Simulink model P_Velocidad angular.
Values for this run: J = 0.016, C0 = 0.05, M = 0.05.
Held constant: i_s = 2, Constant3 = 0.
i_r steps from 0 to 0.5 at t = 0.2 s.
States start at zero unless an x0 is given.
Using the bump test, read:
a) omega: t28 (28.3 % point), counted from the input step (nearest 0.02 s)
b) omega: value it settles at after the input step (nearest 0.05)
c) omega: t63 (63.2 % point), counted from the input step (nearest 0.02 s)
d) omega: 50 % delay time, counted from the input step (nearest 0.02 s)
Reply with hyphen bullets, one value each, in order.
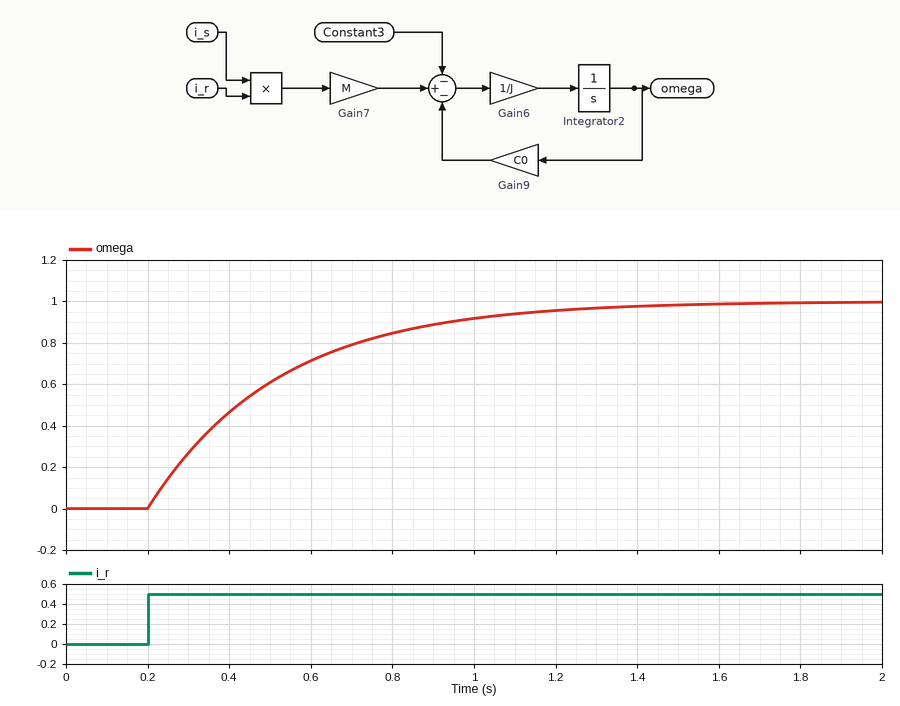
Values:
- 0.10 s
- 1.00
- 0.32 s
- 0.22 s
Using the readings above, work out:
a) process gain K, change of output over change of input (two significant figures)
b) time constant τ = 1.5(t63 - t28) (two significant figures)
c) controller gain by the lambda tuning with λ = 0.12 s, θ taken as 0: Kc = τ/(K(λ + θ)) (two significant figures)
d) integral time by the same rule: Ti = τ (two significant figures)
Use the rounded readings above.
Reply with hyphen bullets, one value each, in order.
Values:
- 2.0
- 0.33 s
- 1.4
- 0.33 s
